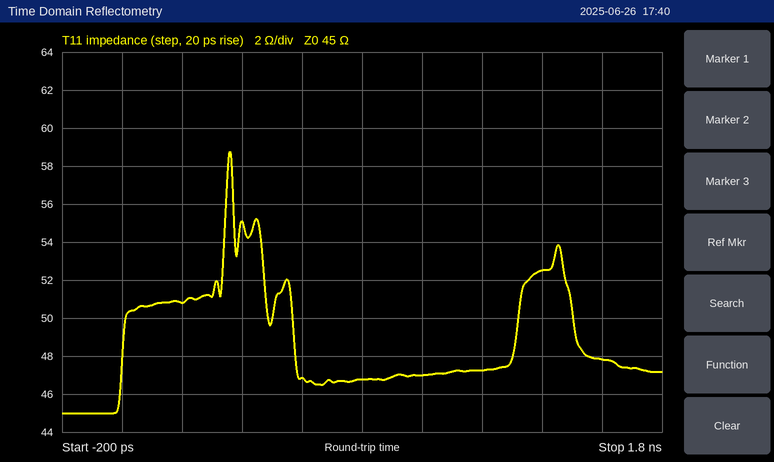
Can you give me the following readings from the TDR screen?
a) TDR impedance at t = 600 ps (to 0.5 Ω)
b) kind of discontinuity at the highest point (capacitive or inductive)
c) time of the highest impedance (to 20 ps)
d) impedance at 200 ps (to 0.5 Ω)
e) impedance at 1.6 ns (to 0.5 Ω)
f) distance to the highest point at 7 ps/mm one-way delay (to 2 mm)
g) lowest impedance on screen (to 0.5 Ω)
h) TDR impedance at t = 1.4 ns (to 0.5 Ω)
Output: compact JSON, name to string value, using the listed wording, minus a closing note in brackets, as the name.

{"TDR impedance at t = 600 ps": "47.0 Ω", "kind of discontinuity at the highest point": "inductive", "time of the highest impedance": "360 ps", "impedance at 200 ps": "51.0 Ω", "impedance at 1.6 ns": "48.0 Ω", "distance to the highest point at 7 ps/mm one-way delay": "26 mm", "lowest impedance on screen": "45.0 Ω", "TDR impedance at t = 1.4 ns": "52.5 Ω"}
